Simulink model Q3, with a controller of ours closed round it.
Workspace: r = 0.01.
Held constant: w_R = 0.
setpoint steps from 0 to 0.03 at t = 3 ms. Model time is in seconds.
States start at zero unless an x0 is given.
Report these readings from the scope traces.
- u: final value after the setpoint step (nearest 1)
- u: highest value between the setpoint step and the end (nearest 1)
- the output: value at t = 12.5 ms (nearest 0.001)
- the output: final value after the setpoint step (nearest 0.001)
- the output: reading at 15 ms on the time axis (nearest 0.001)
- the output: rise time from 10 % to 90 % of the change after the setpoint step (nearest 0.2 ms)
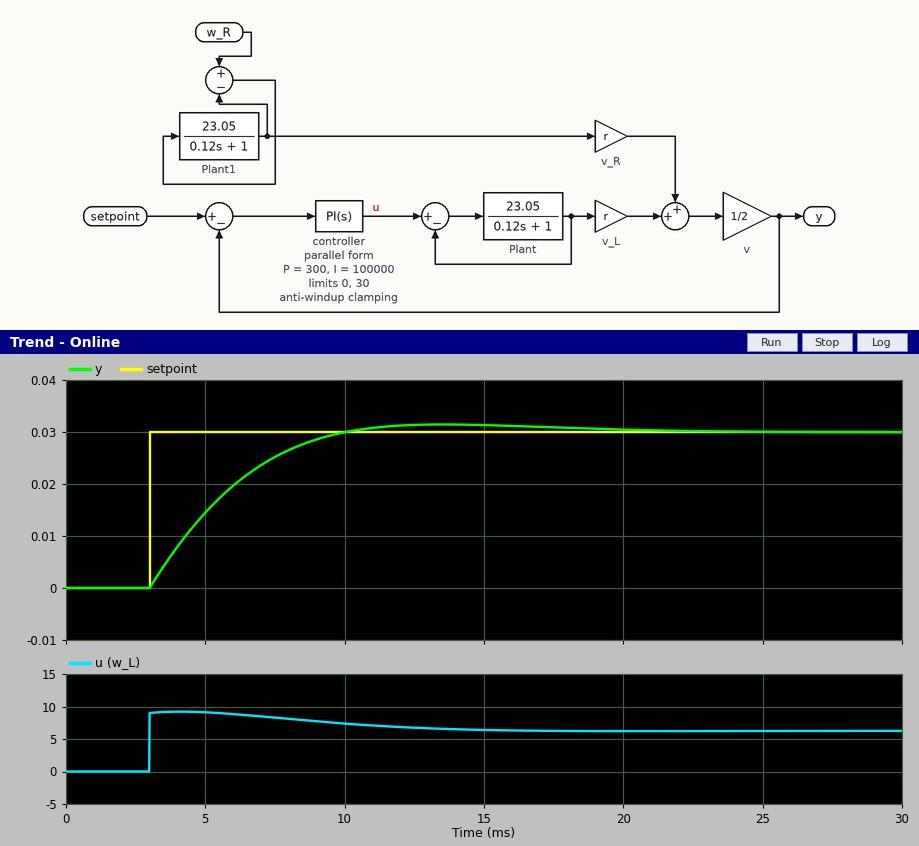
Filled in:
6
9
0.031
0.030
0.031
4.8 ms
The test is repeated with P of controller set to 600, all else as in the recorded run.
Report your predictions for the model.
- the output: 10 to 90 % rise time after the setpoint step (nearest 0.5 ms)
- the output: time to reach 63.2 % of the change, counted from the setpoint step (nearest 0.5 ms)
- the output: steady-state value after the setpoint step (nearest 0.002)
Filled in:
4.5 ms
2.0 ms
0.030
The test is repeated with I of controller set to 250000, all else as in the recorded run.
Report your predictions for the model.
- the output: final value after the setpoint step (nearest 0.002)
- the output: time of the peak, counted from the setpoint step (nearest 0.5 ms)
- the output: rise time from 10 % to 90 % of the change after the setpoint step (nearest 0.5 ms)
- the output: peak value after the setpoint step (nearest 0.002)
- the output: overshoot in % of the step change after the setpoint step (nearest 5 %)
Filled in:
0.030
6.0 ms
2.5 ms
0.036
20 %
